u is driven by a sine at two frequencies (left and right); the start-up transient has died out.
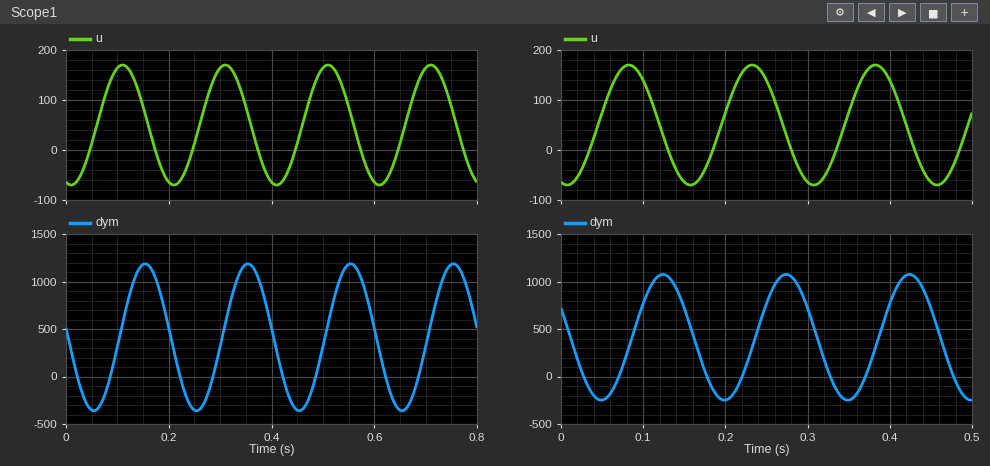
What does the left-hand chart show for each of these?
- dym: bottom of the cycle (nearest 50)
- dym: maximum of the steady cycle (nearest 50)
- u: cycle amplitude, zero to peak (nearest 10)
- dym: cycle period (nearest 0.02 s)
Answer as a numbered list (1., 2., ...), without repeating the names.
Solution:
1. -350
2. 1200
3. 120
4. 0.20 s
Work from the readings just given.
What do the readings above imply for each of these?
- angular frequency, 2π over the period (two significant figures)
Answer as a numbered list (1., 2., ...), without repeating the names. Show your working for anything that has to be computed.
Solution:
1. 2π / 0.2 = 31 rad/s
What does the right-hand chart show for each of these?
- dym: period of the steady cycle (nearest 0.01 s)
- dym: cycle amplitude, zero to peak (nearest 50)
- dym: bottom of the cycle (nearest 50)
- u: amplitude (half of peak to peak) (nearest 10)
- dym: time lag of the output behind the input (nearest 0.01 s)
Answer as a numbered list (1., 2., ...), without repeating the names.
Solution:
1. 0.15 s
2. 650
3. -250
4. 120
5. 0.04 s
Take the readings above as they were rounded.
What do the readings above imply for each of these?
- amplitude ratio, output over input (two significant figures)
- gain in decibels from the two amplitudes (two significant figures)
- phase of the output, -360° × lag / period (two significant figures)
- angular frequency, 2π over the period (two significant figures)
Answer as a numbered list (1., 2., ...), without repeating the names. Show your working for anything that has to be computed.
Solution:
1. 650 / 120 = 5.4
2. 20 log10(650 / 120) = 15 dB
3. -360 × 0.04 / 0.15 = -96°
4. 2π / 0.15 = 42 rad/s
